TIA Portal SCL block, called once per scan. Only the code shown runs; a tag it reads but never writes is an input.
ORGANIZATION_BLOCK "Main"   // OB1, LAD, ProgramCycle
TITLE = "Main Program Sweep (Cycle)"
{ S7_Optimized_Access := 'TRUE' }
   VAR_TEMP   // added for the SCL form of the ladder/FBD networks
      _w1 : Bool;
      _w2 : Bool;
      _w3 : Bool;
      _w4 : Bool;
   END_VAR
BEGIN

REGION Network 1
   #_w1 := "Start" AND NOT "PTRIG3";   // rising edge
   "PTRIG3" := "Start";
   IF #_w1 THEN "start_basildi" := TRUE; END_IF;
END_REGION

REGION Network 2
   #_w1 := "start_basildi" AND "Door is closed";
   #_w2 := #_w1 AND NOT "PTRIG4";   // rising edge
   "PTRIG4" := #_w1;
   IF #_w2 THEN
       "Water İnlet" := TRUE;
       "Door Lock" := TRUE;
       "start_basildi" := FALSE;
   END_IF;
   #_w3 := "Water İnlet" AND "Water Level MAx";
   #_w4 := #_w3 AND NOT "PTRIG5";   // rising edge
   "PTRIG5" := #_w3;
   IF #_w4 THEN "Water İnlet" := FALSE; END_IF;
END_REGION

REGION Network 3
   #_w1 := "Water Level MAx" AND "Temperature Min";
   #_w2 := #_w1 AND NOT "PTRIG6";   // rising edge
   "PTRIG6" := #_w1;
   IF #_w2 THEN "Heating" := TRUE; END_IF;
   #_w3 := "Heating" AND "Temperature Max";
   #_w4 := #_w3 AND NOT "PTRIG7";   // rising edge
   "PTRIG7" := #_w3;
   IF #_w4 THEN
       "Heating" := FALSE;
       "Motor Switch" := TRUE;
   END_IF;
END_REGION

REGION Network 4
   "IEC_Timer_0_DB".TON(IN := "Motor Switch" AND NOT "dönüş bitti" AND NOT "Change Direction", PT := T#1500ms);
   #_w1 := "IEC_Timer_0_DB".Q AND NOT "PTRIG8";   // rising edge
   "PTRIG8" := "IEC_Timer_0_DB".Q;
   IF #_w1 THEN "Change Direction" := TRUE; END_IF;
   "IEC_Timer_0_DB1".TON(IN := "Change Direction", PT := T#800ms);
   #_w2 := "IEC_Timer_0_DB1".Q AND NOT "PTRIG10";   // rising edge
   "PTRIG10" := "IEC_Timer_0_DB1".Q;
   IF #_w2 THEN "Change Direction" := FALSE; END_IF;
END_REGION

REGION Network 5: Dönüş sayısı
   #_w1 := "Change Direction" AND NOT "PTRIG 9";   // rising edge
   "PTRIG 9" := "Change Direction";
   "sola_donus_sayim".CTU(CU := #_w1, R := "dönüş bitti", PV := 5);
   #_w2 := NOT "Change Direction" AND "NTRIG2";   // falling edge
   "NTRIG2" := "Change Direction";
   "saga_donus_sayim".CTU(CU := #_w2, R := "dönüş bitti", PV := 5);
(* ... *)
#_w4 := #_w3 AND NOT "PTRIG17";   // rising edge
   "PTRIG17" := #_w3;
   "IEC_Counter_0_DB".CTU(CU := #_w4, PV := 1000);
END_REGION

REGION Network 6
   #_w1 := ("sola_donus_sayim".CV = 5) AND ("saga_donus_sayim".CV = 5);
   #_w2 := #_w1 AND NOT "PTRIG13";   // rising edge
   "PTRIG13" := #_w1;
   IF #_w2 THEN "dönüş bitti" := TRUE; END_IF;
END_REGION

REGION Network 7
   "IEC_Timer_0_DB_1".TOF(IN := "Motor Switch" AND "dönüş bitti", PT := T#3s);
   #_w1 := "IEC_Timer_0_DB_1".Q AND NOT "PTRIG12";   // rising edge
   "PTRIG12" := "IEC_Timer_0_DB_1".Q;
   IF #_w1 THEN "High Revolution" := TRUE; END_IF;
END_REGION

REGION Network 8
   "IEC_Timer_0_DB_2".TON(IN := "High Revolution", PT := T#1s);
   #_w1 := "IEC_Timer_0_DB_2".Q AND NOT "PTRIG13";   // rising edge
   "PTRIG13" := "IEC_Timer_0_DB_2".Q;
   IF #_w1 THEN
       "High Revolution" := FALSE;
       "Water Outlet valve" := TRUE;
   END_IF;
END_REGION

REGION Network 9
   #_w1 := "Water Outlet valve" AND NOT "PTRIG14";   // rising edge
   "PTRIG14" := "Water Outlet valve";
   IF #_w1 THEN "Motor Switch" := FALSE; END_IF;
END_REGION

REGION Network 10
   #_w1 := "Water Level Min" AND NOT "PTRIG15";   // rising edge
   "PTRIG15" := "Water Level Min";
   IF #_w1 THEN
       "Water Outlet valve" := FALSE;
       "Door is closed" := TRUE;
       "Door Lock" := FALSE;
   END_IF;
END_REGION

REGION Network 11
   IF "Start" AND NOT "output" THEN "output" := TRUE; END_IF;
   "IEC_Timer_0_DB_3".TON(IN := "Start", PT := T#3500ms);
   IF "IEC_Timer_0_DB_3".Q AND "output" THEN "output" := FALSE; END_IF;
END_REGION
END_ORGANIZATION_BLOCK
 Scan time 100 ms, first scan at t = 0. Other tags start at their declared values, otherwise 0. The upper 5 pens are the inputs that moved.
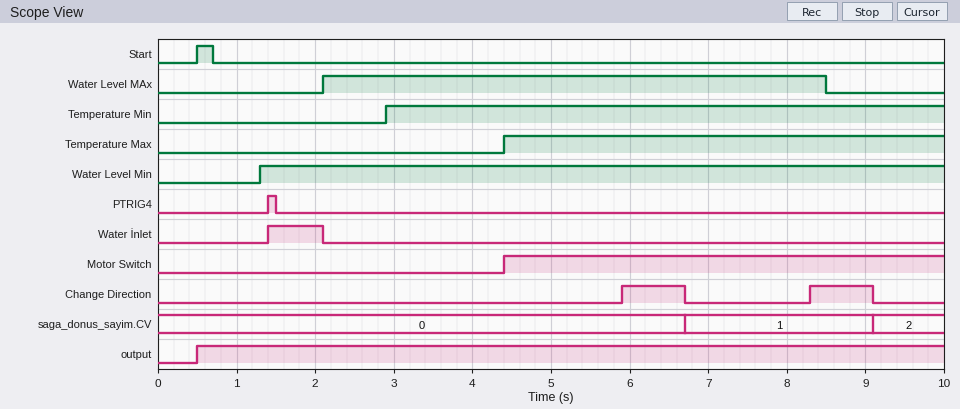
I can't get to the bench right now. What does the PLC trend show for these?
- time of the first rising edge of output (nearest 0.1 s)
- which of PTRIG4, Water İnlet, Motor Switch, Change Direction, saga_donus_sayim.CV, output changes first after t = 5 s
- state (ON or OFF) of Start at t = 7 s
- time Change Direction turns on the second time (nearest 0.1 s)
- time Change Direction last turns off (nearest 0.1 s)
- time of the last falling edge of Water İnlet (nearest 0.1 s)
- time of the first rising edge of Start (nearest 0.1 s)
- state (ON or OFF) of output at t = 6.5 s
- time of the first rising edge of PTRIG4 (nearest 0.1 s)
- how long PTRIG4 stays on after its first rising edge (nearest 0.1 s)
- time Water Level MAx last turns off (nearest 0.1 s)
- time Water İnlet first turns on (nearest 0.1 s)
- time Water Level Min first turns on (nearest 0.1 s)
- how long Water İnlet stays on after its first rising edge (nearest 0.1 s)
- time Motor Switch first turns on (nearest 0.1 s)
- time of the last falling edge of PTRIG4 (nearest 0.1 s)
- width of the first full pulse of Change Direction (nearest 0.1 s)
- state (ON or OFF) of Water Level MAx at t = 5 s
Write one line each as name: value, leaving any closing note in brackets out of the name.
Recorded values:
time of the first rising edge of output: 0.5 s
which of PTRIG4, Water İnlet, Motor Switch, Change Direction, saga_donus_sayim.CV, output changes first after t = 5 s: Change Direction
state (ON or OFF) of Start at t = 7 s: OFF
time Change Direction turns on the second time: 8.3 s
time Change Direction last turns off: 9.1 s
time of the last falling edge of Water İnlet: 2.1 s
time of the first rising edge of Start: 0.5 s
state (ON or OFF) of output at t = 6.5 s: ON
time of the first rising edge of PTRIG4: 1.4 s
how long PTRIG4 stays on after its first rising edge: 0.1 s
time Water Level MAx last turns off: 8.5 s
time Water İnlet first turns on: 1.4 s
time Water Level Min first turns on: 1.3 s
how long Water İnlet stays on after its first rising edge: 0.7 s
time Motor Switch first turns on: 4.4 s
time of the last falling edge of PTRIG4: 1.5 s
width of the first full pulse of Change Direction: 0.8 s
state (ON or OFF) of Water Level MAx at t = 5 s: ON
